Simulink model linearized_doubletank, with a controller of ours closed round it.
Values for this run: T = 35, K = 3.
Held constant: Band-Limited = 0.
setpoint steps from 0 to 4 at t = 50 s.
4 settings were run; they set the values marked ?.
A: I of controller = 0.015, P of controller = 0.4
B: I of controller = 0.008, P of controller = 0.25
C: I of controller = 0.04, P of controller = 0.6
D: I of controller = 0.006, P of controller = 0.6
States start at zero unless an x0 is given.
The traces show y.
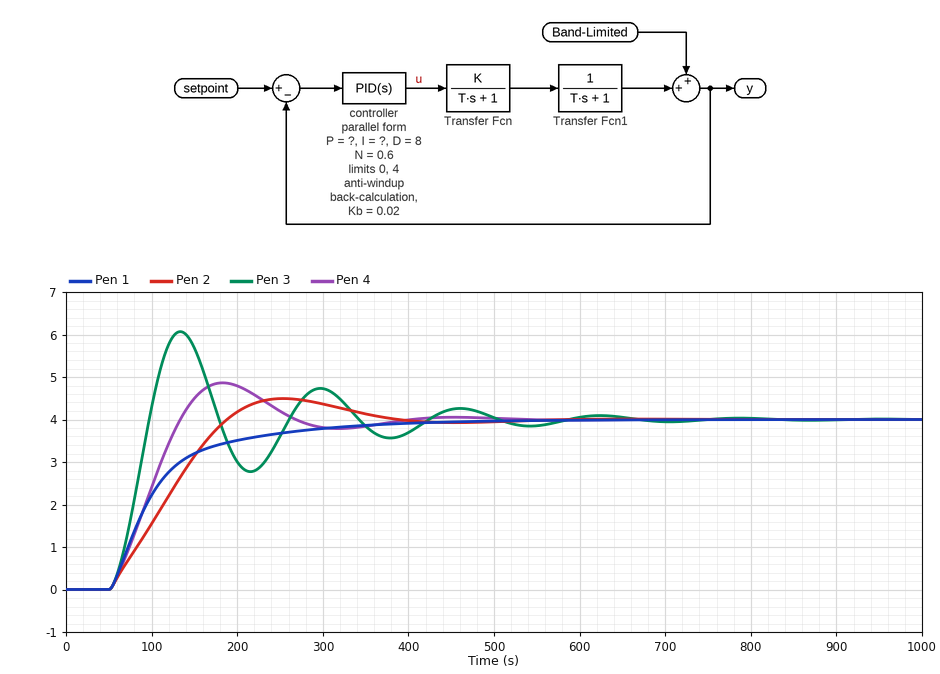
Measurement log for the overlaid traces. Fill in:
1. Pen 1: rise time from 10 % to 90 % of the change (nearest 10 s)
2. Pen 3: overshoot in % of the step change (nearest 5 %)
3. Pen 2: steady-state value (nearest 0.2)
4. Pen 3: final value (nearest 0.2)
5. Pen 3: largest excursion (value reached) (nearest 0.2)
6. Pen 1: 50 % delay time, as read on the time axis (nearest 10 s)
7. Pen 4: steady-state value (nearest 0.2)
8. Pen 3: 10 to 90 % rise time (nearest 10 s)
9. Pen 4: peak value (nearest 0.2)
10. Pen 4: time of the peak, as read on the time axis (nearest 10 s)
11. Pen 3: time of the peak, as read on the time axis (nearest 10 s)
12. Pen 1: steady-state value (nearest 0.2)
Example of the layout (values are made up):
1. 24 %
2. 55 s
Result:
1. 160 s
2. 50 %
3. 4.0
4. 4.0
5. 6.0
6. 90 s
7. 4.0
8. 30 s
9. 4.8
10. 180 s
11. 130 s
12. 4.0
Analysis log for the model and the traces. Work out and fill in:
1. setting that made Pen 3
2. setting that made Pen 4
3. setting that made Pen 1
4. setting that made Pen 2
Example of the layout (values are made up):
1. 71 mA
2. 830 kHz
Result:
1. C
2. A
3. D
4. B
